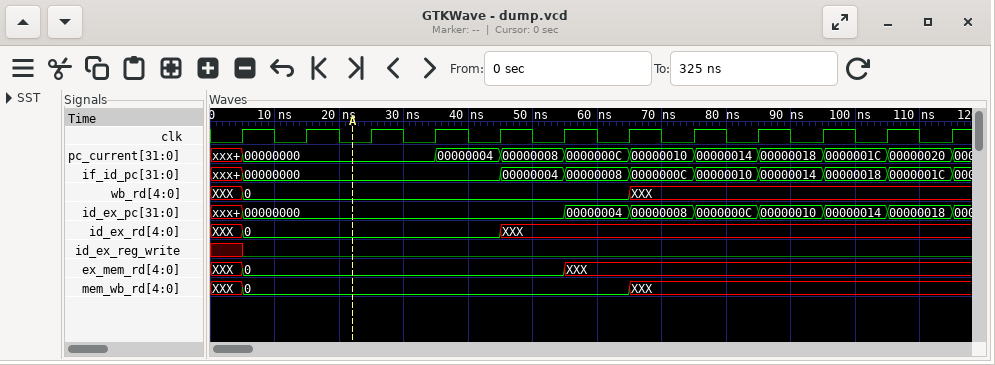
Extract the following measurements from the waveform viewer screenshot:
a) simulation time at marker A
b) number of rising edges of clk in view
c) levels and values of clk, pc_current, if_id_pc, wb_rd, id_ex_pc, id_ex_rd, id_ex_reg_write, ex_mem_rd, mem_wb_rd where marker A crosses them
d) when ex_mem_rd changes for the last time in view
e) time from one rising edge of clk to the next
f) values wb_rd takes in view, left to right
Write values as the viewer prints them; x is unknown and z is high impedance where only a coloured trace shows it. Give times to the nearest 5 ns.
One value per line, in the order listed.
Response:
20 ns
12
clk=0, pc_current=00000000, if_id_pc=00000000, wb_rd=0, id_ex_pc=00000000, id_ex_rd=0, id_ex_reg_write=0, ex_mem_rd=0, mem_wb_rd=0
55 ns
10 ns
XXX, 0, XXX
